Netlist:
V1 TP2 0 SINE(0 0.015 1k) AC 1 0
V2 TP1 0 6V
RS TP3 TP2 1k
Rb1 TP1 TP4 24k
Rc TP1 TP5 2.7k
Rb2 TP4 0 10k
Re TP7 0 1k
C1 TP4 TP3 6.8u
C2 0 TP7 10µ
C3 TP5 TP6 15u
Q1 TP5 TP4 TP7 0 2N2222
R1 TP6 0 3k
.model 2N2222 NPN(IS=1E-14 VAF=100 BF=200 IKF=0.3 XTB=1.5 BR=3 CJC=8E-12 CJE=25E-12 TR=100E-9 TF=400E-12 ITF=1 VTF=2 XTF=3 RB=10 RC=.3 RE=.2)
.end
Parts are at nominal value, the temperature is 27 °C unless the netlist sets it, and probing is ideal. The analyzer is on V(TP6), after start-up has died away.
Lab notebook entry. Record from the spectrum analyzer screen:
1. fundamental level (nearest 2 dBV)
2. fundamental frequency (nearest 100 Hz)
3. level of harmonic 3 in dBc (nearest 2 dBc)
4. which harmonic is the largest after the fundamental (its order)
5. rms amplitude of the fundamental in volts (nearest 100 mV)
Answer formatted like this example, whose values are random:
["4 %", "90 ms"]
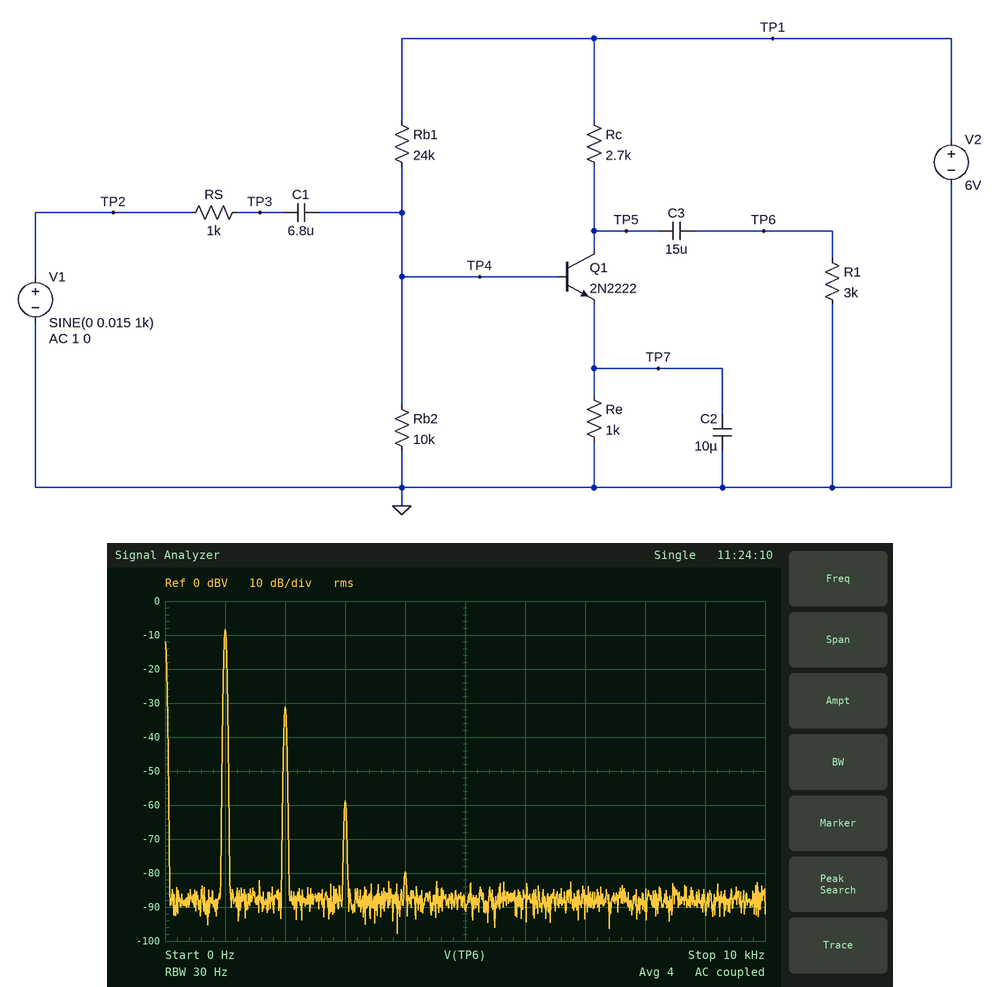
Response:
["-8 dBV", "1.0 kHz", "-50 dBc", "2", "400 mV"]
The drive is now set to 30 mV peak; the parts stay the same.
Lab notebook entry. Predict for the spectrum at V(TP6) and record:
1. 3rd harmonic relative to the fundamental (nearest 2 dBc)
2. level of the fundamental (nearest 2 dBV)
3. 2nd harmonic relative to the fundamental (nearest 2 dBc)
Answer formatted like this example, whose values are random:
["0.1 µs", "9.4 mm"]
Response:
["-38 dBc", "-2 dBV", "-16 dBc"]
